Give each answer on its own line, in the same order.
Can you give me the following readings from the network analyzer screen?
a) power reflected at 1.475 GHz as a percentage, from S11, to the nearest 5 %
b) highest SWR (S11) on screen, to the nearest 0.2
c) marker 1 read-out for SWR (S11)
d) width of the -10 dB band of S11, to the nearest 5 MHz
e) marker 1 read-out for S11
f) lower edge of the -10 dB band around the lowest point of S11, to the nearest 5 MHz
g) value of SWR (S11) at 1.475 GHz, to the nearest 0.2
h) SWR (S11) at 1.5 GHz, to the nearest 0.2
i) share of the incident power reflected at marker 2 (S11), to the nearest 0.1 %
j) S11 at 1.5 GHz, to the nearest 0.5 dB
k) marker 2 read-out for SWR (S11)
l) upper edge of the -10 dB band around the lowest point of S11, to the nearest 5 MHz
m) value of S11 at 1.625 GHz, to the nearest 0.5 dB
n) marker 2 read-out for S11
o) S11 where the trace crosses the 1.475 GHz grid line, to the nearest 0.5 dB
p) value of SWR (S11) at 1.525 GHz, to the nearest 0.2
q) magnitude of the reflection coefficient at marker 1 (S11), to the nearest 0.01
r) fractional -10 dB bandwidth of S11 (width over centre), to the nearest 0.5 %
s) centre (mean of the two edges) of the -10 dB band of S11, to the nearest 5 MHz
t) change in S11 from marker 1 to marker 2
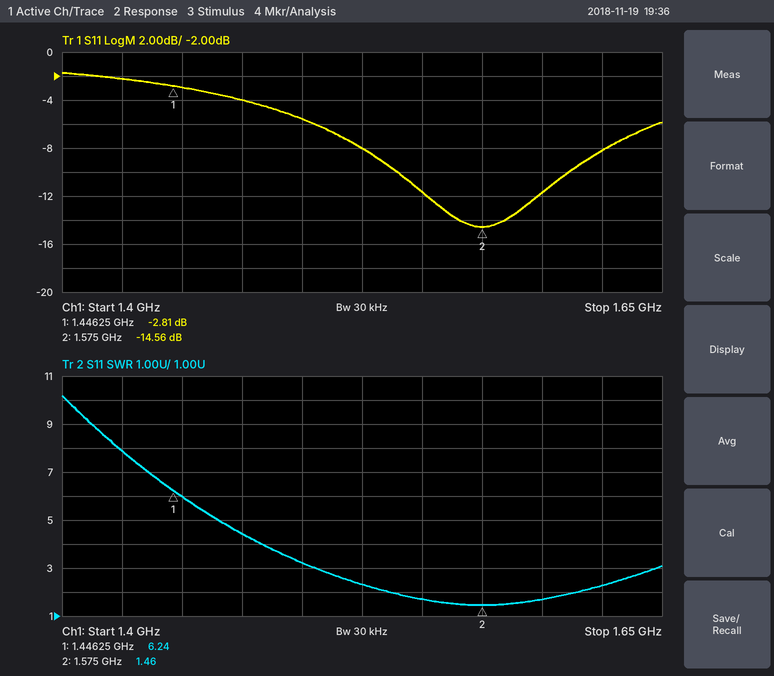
40 %
10.2
6.24
70 MHz
-2.81 dB
1.540 GHz
4.4
3.2
3.5 %
-5.5 dB
1.46
1.610 GHz
-8.0 dB
-14.56 dB
-4.0 dB
2.4
0.72
4.5 %
1.575 GHz
-11.75 dB
